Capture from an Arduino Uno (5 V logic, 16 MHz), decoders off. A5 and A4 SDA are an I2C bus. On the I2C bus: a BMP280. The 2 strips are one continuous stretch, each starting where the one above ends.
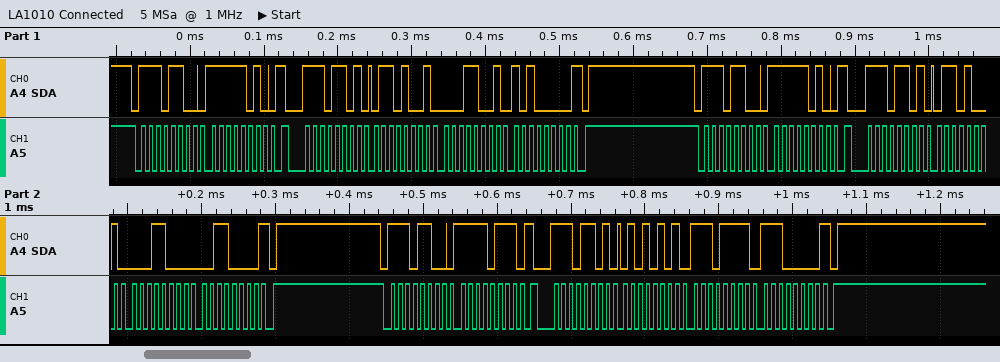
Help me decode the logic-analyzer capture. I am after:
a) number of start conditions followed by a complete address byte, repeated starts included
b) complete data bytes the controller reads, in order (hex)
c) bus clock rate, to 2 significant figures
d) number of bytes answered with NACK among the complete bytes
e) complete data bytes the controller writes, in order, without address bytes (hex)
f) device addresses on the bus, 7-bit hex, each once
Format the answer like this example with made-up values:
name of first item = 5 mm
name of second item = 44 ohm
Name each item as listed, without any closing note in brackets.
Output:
number of start conditions followed by a complete address byte, repeated starts included = 6
complete data bytes the controller reads, in order = 69 19 A0 69 18 30 55 EF E0
bus clock rate, to 2 significant figures = 100 kHz
number of bytes answered with NACK among the complete bytes = 3
complete data bytes the controller writes, in order, without address bytes = FA FA F7
device addresses on the bus, 7-bit hex, each once = 0x76
